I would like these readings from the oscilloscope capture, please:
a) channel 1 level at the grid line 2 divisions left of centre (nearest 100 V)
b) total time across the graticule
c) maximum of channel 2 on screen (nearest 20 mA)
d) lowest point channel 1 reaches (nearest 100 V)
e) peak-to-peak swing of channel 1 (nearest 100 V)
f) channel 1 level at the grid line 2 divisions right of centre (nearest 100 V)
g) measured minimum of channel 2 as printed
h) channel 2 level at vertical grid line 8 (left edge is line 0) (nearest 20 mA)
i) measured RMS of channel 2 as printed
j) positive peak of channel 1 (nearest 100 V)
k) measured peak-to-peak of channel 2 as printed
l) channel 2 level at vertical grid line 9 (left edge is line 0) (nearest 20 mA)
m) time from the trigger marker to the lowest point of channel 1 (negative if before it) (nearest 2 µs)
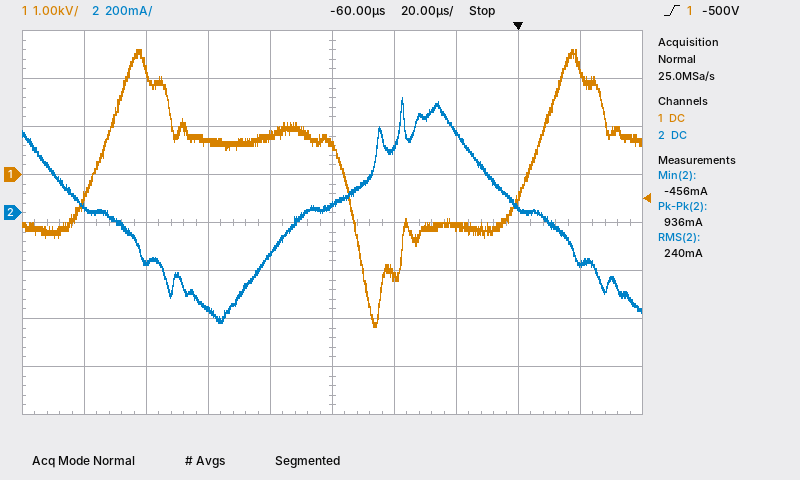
700 V
200 µs
480 mA
-3.2 kV
5.8 kV
-1.1 kV
-456 mA
20 mA
240 mA
2.6 kV
936 mA
-220 mA
-46 µs
